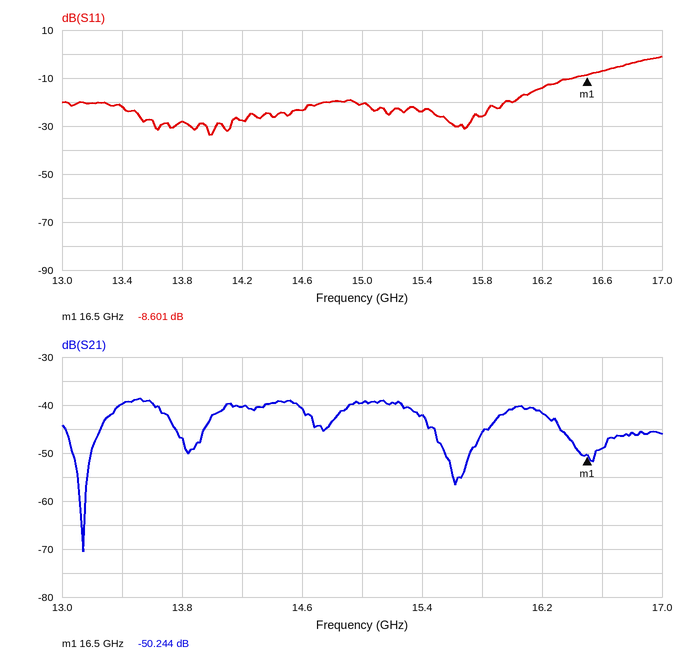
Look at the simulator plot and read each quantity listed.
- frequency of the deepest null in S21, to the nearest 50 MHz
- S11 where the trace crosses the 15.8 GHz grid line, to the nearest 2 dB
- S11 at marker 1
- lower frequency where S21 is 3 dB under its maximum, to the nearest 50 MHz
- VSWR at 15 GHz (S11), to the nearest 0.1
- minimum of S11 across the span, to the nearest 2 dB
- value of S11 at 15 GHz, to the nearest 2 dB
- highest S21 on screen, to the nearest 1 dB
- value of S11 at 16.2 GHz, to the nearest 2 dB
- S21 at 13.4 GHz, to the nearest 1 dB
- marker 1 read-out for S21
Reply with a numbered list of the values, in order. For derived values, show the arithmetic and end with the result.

1. 13.15 GHz
2. -26 dB
3. -8.601 dB
4. 13.35 GHz
5. |Γ| = 10^(-20/20) = 0.1000; VSWR = (1 + 0.1000)/(1 − 0.1000) ≈ 1.2
6. -34 dB
7. -20 dB
8. -39 dB
9. -14 dB
10. -40 dB
11. -50.244 dB
